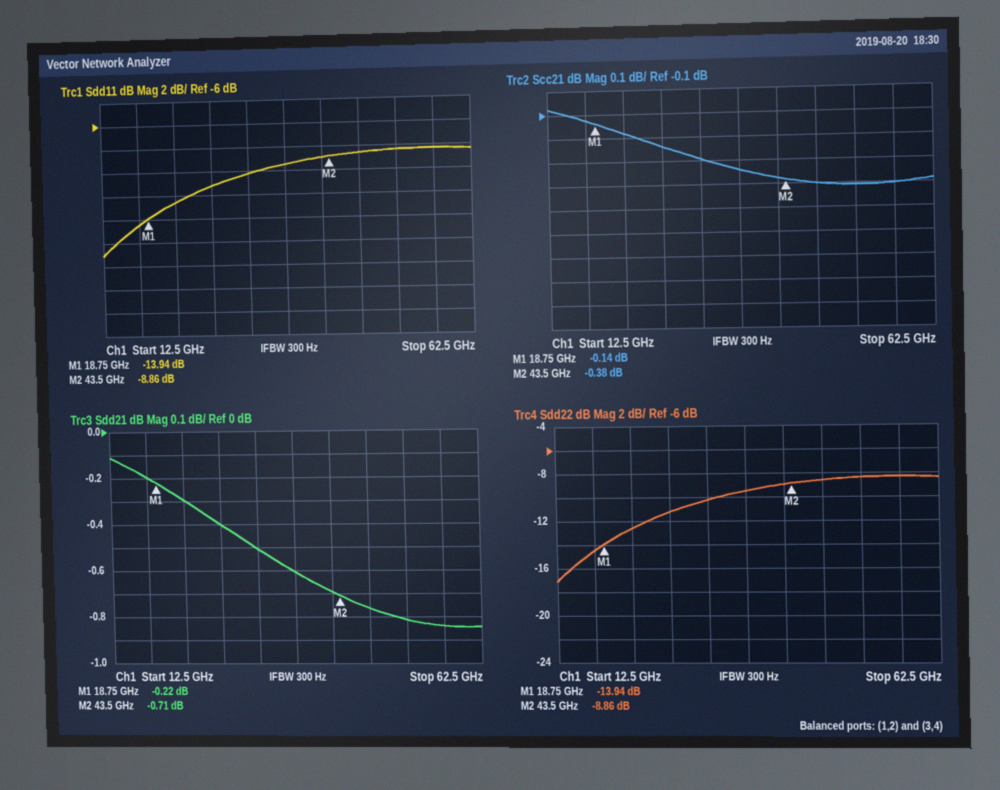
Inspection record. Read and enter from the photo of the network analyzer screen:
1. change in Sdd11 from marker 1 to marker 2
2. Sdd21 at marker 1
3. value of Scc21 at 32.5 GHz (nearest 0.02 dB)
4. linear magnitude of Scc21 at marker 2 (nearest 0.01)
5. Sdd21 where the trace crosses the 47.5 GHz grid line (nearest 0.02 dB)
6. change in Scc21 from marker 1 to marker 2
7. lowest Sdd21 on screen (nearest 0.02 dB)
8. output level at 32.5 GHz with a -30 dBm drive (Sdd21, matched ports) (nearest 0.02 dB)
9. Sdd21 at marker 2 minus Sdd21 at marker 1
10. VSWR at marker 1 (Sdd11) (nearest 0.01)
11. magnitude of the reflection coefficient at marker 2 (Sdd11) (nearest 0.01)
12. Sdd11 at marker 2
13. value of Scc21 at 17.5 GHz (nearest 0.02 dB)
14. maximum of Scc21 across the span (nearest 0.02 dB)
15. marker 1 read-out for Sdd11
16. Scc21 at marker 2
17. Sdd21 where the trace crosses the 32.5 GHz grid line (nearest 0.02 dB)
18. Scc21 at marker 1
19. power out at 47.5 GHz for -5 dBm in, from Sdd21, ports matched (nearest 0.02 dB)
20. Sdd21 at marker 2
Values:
5.08 dB
-0.22 dB
-0.30 dB
0.96
-0.76 dB
-0.24 dB
-0.84 dB
-30.50 dBm
-0.49 dB
1.50
0.36
-8.86 dB
-0.12 dB
-0.08 dB
-13.94 dB
-0.38 dB
-0.50 dB
-0.14 dB
-5.76 dBm
-0.71 dB
